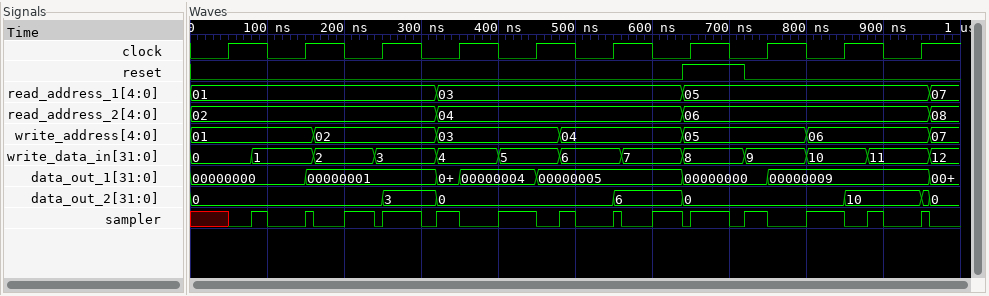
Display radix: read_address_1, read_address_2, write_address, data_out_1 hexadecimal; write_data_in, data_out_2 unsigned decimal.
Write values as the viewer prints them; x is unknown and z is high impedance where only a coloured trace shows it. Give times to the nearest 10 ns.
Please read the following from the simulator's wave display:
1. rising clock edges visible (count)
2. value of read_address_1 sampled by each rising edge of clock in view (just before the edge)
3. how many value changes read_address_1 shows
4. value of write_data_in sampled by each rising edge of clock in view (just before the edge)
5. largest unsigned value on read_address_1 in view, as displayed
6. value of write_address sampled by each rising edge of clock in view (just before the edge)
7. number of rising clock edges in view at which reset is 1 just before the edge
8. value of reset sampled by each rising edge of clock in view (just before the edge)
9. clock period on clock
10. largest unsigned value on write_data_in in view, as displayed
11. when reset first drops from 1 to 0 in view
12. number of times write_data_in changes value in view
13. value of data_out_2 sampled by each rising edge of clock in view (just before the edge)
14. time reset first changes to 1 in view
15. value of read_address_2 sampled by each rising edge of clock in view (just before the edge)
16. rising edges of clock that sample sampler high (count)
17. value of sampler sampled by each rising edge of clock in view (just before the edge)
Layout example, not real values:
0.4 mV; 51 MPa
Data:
10; 01, 01, 01, 03, 03, 03, 05, 05, 05, 05; 3; 0, 1, 3, 4, 5, 6, 8, 9, 10, 11; 07; 01, 01, 02, 03, 03, 04, 05, 05, 06, 06; 1; 0 0 0 0 0 0 1 0 0 0; 100 ns; 12; 720 ns; 12; 0, 0, 0, 0, 0, 0, 0, 0, 0, 10; 640 ns; 02, 02, 02, 04, 04, 04, 06, 06, 06, 06; 4; x 0 0 1 1 0 0 1 1 0
